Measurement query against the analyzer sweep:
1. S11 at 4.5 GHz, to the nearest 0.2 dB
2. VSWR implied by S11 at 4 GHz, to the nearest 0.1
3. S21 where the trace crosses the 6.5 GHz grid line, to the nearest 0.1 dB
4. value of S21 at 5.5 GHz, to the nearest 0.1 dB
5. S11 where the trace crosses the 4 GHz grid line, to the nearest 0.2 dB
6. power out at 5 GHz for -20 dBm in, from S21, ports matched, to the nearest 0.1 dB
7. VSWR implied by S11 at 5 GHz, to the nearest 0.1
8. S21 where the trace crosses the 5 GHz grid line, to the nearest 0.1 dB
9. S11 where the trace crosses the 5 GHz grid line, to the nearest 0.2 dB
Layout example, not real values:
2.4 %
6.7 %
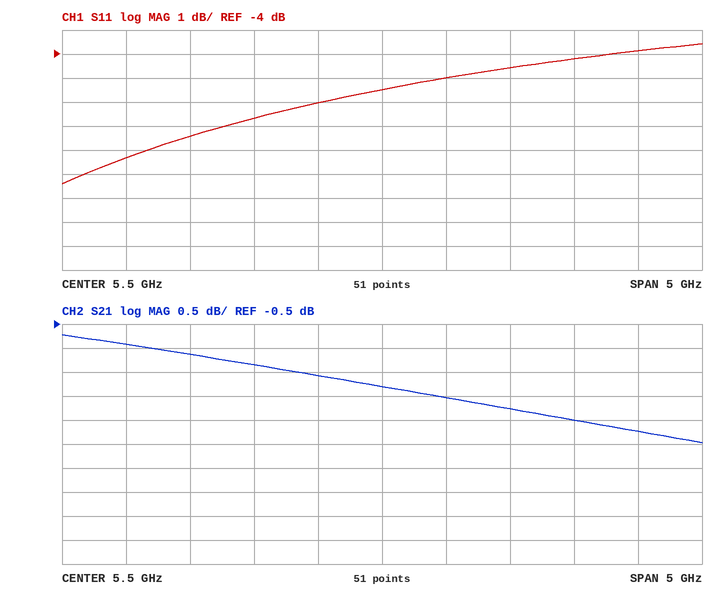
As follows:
-6.6 dB
2.5
-2.3 dB
-1.8 dB
-7.4 dB
-21.6 dBm
3.0
-1.6 dB
-6.0 dB
